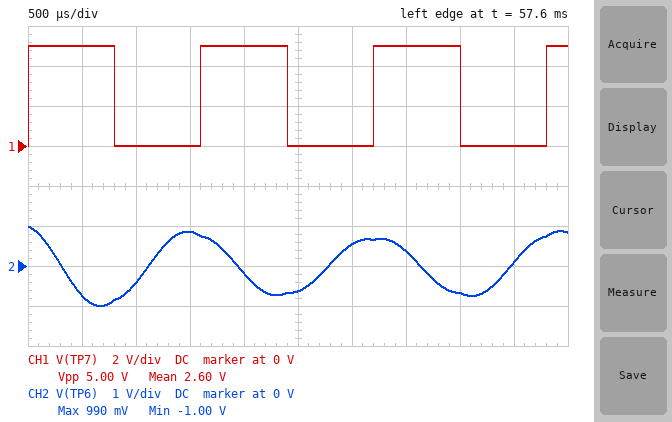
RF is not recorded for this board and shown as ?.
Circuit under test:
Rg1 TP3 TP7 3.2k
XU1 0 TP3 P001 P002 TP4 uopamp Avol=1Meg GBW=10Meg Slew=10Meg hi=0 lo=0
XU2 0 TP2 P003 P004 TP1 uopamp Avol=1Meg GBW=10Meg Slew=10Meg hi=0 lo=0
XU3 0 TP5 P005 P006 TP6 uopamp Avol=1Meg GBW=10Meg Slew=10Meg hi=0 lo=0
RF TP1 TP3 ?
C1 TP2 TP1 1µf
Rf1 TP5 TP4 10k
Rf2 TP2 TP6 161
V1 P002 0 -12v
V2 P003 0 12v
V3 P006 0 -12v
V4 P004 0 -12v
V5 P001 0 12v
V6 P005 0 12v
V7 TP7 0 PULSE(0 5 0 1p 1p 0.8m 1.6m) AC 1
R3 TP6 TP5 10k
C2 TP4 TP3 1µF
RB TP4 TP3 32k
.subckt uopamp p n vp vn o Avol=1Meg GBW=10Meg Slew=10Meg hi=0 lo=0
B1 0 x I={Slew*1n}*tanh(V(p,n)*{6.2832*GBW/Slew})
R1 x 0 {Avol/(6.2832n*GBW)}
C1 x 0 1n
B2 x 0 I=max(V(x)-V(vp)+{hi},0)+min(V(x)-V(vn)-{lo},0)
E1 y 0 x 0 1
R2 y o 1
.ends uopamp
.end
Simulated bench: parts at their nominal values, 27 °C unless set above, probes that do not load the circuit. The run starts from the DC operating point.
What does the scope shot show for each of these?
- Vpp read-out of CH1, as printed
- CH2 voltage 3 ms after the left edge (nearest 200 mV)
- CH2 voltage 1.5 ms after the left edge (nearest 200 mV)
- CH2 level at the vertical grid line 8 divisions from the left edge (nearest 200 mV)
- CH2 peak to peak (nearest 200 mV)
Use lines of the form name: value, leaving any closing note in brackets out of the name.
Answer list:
Vpp read-out of CH1, as printed: 5.00 V
CH2 voltage 3 ms after the left edge: 600 mV
CH2 voltage 1.5 ms after the left edge: 800 mV
CH2 level at the vertical grid line 8 divisions from the left edge: -600 mV
CH2 peak to peak: 2.0 V
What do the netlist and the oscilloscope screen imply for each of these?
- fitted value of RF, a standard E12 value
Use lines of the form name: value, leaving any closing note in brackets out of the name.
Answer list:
fitted value of RF, a standard E12 value: 330 Ω
